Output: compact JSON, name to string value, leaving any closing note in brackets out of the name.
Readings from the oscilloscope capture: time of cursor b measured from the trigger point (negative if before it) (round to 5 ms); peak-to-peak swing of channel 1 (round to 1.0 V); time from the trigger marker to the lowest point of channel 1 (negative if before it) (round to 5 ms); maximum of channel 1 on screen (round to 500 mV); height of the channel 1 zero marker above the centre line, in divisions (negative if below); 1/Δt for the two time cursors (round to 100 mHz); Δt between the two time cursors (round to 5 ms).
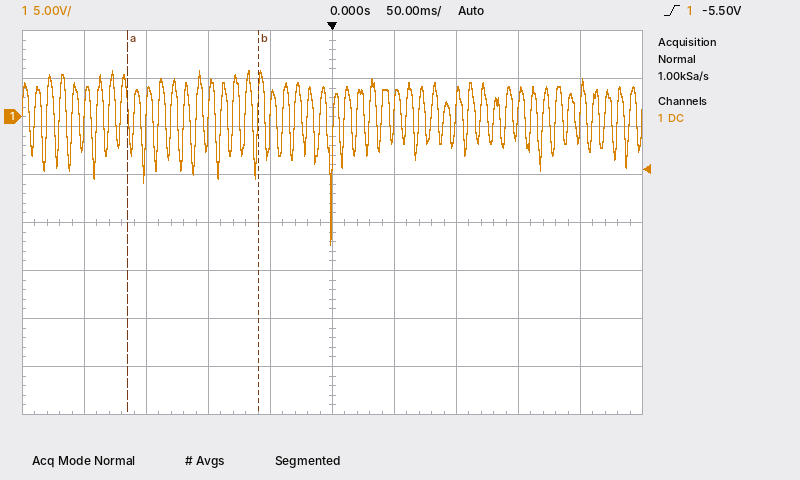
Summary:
{"time of cursor b measured from the trigger point (negative if before it)": "-60 ms", "peak-to-peak swing of channel 1": "18.0 V", "time from the trigger marker to the lowest point of channel 1 (negative if before it)": "0 ms", "maximum of channel 1 on screen": "5.0 V", "height of the channel 1 zero marker above the centre line, in divisions": "+2.2 div", "1/Δt for the two time cursors": "9.5 Hz", "Δt between the two time cursors": "105 ms"}
